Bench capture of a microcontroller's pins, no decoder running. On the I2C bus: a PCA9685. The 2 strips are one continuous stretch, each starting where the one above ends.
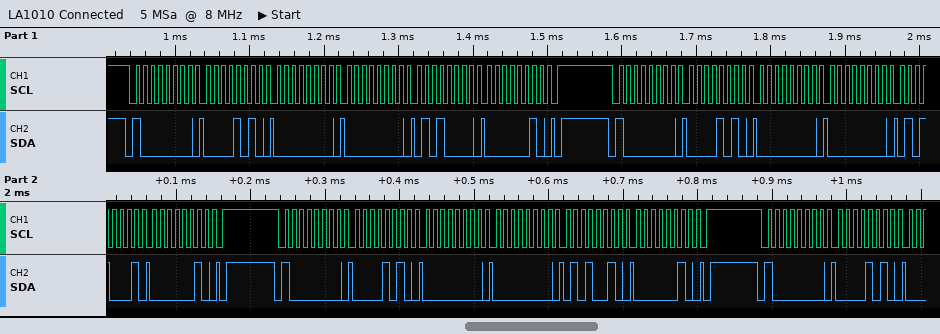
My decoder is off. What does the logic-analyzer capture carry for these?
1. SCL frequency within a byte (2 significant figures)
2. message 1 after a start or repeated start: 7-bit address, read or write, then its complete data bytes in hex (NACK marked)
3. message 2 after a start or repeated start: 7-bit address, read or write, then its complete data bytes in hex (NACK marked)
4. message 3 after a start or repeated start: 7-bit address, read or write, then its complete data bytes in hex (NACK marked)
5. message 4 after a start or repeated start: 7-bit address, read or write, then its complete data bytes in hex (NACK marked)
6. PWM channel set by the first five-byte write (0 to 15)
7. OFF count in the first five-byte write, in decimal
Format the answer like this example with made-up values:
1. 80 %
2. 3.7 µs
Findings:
1. 100 kHz
2. 0x40 write: 0A 00 00 50 02
3. 0x40 write: 0A 00 00 51 02
4. 0x40 write: 0A 00 00 52 02
5. 0x40 write: 0A
6. 1
7. 592
